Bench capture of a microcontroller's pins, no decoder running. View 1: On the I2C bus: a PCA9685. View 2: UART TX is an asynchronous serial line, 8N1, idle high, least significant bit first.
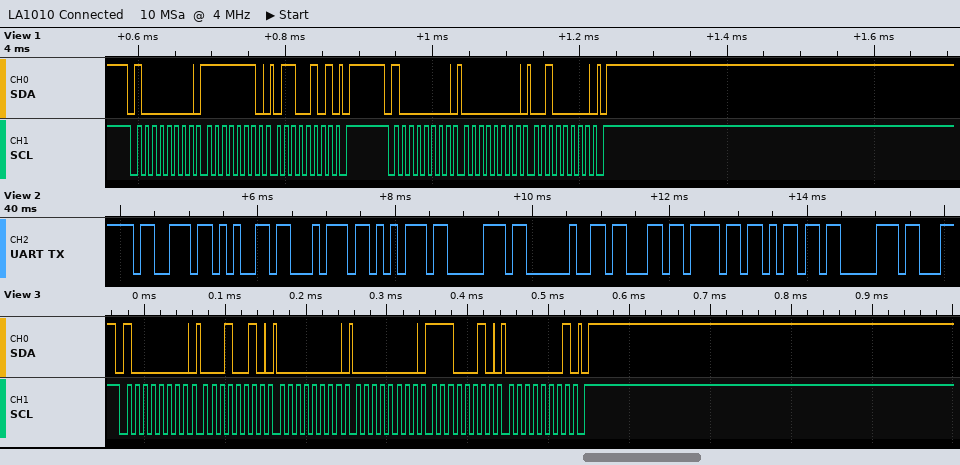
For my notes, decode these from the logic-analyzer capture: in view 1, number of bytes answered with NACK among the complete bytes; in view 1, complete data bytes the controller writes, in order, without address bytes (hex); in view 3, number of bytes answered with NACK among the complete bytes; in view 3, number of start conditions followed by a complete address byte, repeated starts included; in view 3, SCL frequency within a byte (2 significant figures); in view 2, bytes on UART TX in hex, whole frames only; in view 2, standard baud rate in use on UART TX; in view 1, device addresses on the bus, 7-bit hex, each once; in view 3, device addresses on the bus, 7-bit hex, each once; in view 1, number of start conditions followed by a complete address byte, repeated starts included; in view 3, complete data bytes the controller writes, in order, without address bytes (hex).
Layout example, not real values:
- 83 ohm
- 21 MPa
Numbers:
- 0
- FE 65 00 20
- 0
- 1
- 100 kHz
- 0x73 0x65 0x74 0x75 0x70 0x20 0x63 0x6F 0x6D 0x70
- 9600 baud
- 0x40
- 0x40
- 2
- 12 00 00 E2 01
